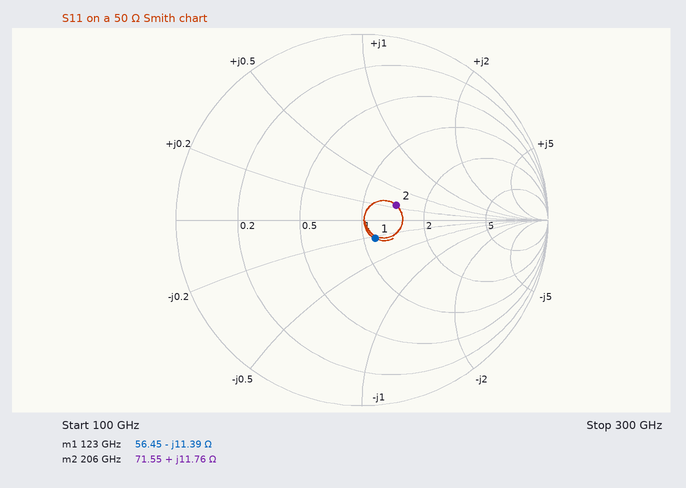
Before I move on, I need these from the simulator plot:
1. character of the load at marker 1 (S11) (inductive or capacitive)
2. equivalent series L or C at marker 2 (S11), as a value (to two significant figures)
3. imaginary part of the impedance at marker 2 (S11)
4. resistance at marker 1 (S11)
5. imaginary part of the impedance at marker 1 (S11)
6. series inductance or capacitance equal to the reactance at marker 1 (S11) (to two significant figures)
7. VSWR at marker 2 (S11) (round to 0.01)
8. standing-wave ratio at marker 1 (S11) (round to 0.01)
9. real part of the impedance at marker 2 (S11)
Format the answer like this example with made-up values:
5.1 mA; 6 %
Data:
capacitive; 9.1 pH; +11.76 Ω; 56.45 Ω; -11.39 Ω; 110 fF; 1.50; 1.28; 71.55 Ω
